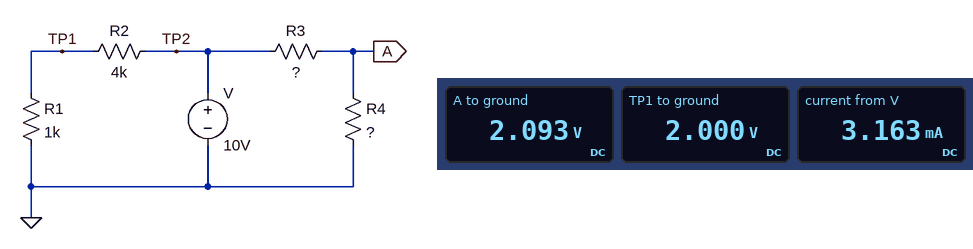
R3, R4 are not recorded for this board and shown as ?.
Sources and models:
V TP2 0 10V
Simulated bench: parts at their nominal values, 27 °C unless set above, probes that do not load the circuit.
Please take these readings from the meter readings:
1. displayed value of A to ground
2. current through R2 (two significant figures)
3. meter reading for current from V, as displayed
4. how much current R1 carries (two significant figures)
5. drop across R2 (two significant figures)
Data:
2.093 V
2.0 mA
3.163 mA
2.0 mA
8.0 V
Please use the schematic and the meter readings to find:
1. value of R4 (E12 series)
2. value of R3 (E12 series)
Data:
1.8 kΩ
6.8 kΩ
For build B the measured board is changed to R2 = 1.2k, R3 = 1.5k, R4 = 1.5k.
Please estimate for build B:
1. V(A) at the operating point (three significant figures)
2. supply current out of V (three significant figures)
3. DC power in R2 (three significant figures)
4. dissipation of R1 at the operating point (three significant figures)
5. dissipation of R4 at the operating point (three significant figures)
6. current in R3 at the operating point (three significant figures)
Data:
5.00 V
7.88 mA
24.8 mW
20.7 mW
16.7 mW
3.33 mA
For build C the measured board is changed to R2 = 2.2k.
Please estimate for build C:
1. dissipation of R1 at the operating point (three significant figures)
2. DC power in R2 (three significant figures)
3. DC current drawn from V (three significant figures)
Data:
9.77 mW
21.5 mW
4.29 mA
